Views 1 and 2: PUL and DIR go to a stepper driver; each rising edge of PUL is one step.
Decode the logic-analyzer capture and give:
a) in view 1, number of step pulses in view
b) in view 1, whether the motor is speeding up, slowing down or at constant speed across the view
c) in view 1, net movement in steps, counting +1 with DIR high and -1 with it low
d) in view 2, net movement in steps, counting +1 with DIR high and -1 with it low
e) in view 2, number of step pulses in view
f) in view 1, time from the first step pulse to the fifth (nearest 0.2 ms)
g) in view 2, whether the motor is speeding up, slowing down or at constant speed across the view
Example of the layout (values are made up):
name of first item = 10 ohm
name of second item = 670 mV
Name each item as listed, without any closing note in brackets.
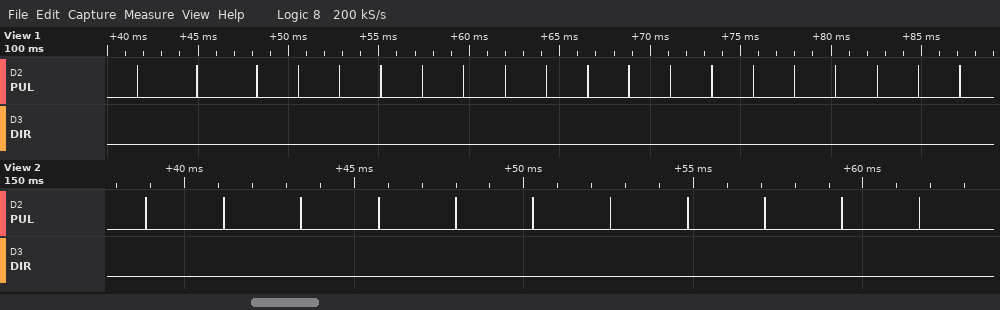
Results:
in view 1, number of step pulses in view = 20
in view 1, whether the motor is speeding up, slowing down or at constant speed across the view = speeding up
in view 1, net movement in steps, counting +1 with DIR high and -1 with it low = -20
in view 2, net movement in steps, counting +1 with DIR high and -1 with it low = -11
in view 2, number of step pulses in view = 11
in view 1, time from the first step pulse to the fifth = 11.2 ms
in view 2, whether the motor is speeding up, slowing down or at constant speed across the view = constant speed
